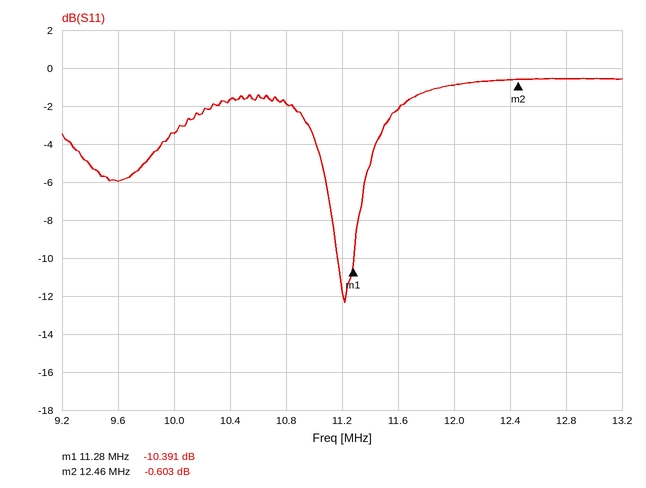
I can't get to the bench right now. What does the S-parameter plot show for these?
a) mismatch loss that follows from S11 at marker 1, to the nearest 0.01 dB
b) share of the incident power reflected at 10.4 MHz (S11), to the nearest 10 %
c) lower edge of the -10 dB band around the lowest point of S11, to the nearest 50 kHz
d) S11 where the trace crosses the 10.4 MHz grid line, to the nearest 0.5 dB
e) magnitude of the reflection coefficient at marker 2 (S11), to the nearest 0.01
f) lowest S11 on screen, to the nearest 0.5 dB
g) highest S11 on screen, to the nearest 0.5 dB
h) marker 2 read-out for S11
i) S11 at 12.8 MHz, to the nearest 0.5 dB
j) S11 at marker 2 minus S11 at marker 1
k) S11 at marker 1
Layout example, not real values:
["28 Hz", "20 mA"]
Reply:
["0.42 dB", "70 %", "11.15 MHz", "-1.5 dB", "0.93", "-12.5 dB", "-0.5 dB", "-0.603 dB", "-0.5 dB", "9.788 dB", "-10.391 dB"]
